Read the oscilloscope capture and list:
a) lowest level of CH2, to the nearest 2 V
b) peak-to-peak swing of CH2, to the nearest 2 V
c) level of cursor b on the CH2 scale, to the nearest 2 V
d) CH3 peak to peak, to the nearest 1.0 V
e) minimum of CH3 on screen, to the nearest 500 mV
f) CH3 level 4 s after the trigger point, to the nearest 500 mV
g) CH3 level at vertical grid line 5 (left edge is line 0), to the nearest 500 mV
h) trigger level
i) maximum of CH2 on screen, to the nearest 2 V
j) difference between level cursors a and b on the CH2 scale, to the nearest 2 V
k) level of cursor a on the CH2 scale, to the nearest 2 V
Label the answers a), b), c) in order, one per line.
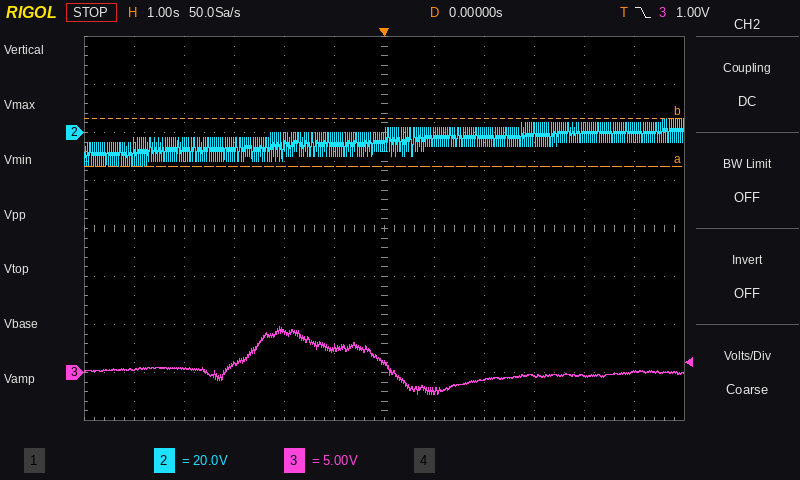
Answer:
a) -14 V
b) 20 V
c) 6 V
d) 7.0 V
e) -2.5 V
f) -500 mV
g) 2.5 V
h) 1.00 V
i) 6 V
j) 20 V
k) -14 V
